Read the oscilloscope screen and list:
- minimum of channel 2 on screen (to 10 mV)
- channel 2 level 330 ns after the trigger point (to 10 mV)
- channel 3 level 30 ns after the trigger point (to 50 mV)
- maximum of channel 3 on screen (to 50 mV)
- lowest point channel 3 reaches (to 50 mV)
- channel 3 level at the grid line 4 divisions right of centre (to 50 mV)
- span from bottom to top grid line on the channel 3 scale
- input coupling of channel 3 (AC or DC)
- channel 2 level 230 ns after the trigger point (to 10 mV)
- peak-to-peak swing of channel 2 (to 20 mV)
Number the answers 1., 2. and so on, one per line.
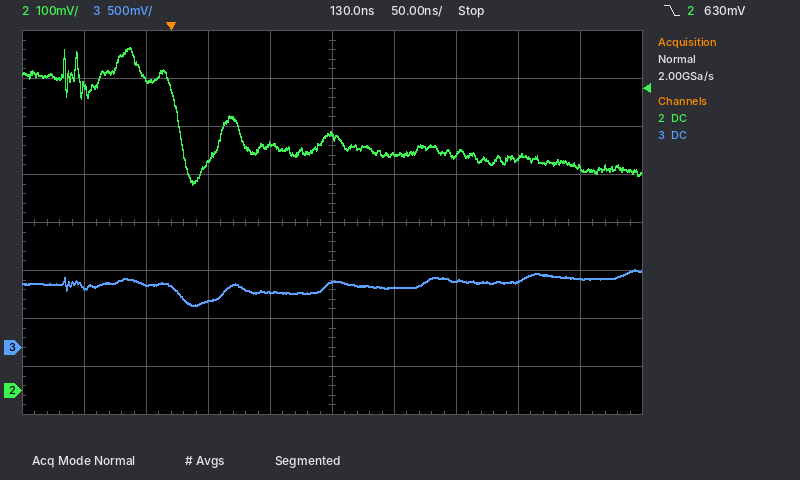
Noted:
1. 430 mV
2. 460 mV
3. 500 mV
4. 800 mV
5. 450 mV
6. 700 mV
7. 4 V
8. DC
9. 490 mV
10. 280 mV
